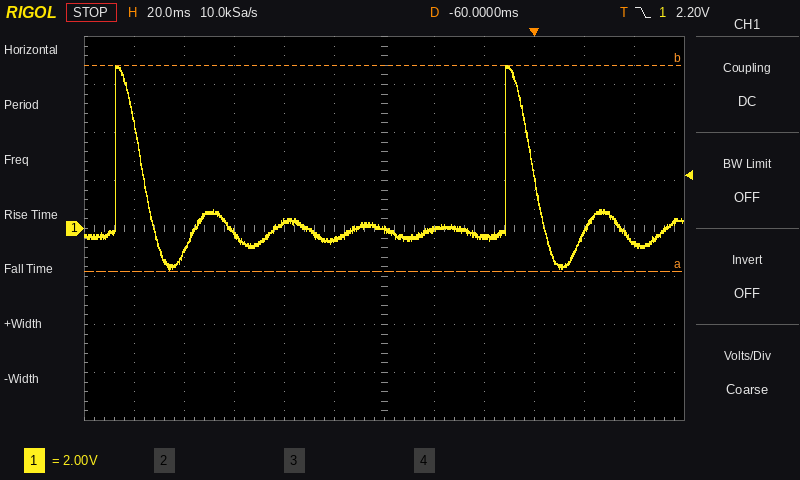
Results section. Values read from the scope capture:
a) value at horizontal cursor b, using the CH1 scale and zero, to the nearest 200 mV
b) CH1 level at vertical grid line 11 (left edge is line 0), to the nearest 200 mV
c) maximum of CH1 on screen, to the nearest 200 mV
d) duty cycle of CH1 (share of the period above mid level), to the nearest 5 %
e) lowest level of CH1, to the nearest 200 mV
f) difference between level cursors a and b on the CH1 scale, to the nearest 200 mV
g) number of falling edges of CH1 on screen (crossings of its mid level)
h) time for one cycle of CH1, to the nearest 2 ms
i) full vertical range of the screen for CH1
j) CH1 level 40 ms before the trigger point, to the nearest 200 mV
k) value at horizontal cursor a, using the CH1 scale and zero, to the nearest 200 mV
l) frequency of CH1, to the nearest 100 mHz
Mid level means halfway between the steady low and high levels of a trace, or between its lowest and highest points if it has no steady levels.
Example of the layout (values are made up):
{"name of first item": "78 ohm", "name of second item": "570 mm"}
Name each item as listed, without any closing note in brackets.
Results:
{"value at horizontal cursor b, using the CH1 scale and zero, to the nearest 200 mV": "6.8 V", "CH1 level at vertical grid line 11 (left edge is line 0), to the nearest 200 mV": "-600 mV", "maximum of CH1 on screen, to the nearest 200 mV": "6.8 V", "duty cycle of CH1 (share of the period above mid level), to the nearest 5 %": "5 %", "lowest level of CH1, to the nearest 200 mV": "-1.8 V", "difference between level cursors a and b on the CH1 scale, to the nearest 200 mV": "8.6 V", "number of falling edges of CH1 on screen": "2", "time for one cycle of CH1, to the nearest 2 ms": "156 ms", "full vertical range of the screen for CH1": "16 V", "CH1 level 40 ms before the trigger point, to the nearest 200 mV": "0.0 V", "value at horizontal cursor a, using the CH1 scale and zero, to the nearest 200 mV": "-1.8 V", "frequency of CH1, to the nearest 100 mHz": "6.4 Hz"}
